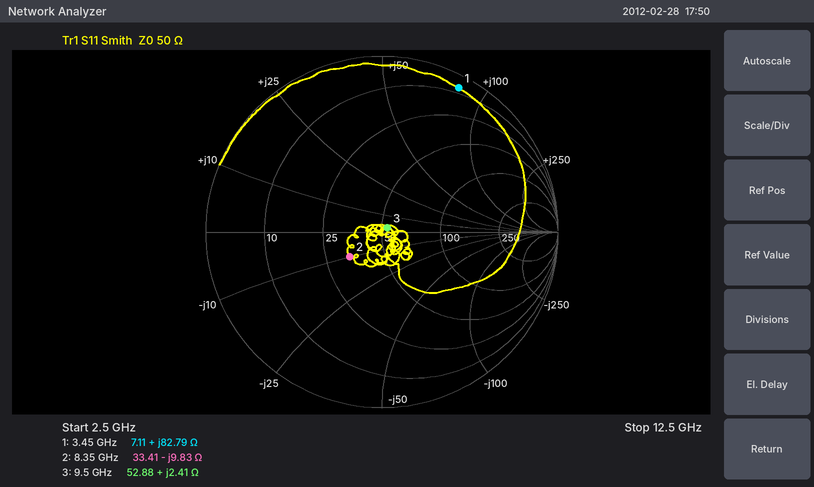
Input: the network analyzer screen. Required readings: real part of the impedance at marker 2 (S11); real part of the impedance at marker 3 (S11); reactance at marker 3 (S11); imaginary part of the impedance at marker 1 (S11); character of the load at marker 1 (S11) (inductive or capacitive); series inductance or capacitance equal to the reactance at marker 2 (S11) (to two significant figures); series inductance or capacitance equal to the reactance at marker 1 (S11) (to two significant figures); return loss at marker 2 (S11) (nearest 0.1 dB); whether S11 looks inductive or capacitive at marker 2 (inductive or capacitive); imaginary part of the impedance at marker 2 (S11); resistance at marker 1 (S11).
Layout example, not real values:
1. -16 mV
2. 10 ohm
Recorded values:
1. 33.41 Ω
2. 52.88 Ω
3. +2.41 Ω
4. +82.79 Ω
5. inductive
6. 1.9 pF
7. 3.8 nH
8. 12.8 dB
9. capacitive
10. -9.83 Ω
11. 7.11 Ω
